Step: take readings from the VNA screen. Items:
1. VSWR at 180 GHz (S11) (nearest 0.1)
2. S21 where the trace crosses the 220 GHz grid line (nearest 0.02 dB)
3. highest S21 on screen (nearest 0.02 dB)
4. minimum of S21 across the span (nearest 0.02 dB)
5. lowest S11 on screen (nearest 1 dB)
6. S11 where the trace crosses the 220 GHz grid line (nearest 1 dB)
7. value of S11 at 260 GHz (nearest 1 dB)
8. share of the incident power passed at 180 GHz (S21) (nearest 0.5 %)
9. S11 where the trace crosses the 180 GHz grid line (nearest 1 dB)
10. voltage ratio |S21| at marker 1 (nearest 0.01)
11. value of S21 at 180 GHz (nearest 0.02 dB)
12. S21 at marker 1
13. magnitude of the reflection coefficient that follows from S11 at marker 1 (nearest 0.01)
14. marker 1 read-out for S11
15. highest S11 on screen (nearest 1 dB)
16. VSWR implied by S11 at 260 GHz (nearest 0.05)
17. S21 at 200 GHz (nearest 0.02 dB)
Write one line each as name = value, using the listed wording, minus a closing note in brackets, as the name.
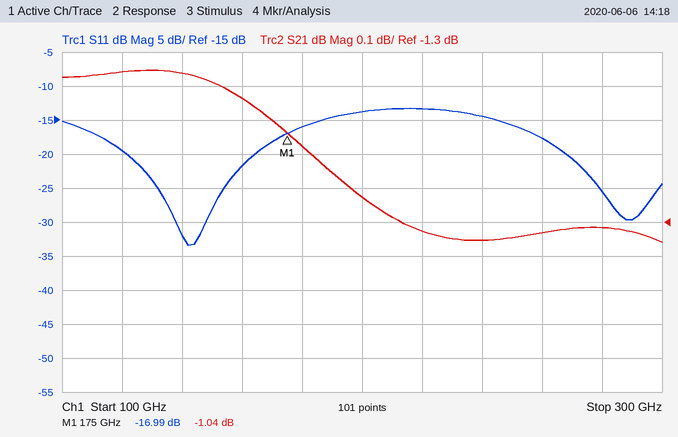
VSWR at 180 GHz (S11) = 1.4
S21 where the trace crosses the 220 GHz grid line = -1.32 dB
highest S21 on screen = -0.86 dB
minimum of S21 across the span = -1.36 dB
lowest S11 on screen = -33 dB
S11 where the trace crosses the 220 GHz grid line = -13 dB
value of S11 at 260 GHz = -18 dB
share of the incident power passed at 180 GHz (S21) = 78.0 %
S11 where the trace crosses the 180 GHz grid line = -16 dB
voltage ratio |S21| at marker 1 = 0.89
value of S21 at 180 GHz = -1.08 dB
S21 at marker 1 = -1.04 dB
magnitude of the reflection coefficient that follows from S11 at marker 1 = 0.14
marker 1 read-out for S11 = -16.99 dB
highest S11 on screen = -13 dB
VSWR implied by S11 at 260 GHz = 1.30
S21 at 200 GHz = -1.22 dB
